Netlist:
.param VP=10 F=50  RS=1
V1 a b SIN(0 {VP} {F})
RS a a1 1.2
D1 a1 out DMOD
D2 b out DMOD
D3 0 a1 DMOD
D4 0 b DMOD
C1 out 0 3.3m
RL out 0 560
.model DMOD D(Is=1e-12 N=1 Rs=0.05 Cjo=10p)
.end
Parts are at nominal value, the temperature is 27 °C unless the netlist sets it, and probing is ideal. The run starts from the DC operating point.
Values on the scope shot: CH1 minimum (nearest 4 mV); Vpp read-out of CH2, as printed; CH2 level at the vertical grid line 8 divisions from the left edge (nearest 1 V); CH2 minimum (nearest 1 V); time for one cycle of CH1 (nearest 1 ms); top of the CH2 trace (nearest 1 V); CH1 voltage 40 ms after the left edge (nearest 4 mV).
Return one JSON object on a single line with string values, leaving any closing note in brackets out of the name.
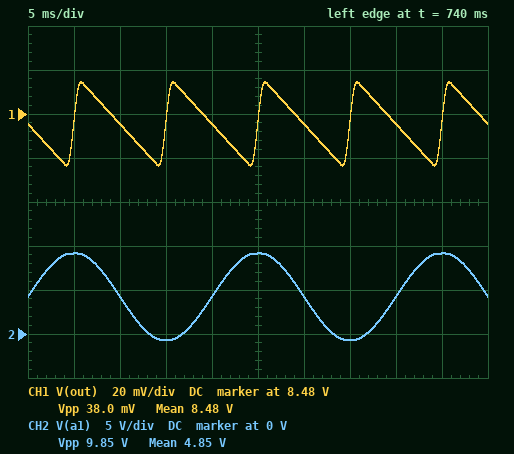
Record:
{"CH1 minimum": "8.456 V", "Vpp read-out of CH2, as printed": "9.85 V", "CH2 level at the vertical grid line 8 divisions from the left edge": "4 V", "CH2 minimum": "-1 V", "time for one cycle of CH1": "10 ms", "top of the CH2 trace": "9 V", "CH1 voltage 40 ms after the left edge": "8.476 V"}
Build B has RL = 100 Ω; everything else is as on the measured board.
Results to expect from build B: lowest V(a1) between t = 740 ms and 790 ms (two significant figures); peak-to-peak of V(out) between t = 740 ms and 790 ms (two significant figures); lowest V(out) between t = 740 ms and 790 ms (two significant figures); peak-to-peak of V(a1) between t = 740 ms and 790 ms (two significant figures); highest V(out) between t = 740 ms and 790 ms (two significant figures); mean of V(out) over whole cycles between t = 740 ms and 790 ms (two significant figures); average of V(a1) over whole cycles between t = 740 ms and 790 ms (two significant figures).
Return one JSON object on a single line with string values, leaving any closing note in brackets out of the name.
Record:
{"lowest V(a1) between t = 740 ms and 790 ms": "-720 mV", "peak-to-peak of V(out) between t = 740 ms and 790 ms": "180 mV", "lowest V(out) between t = 740 ms and 790 ms": "7.9 V", "peak-to-peak of V(a1) between t = 740 ms and 790 ms": "9.5 V", "highest V(out) between t = 740 ms and 790 ms": "8.1 V", "mean of V(out) over whole cycles between t = 740 ms and 790 ms": "8.0 V", "average of V(a1) over whole cycles between t = 740 ms and 790 ms": "4.0 V"}
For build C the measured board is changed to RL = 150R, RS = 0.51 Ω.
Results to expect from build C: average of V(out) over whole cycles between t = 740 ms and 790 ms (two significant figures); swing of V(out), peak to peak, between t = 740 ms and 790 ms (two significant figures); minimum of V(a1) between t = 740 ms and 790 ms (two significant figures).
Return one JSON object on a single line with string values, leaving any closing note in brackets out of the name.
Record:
{"average of V(out) over whole cycles between t = 740 ms and 790 ms": "8.3 V", "swing of V(out), peak to peak, between t = 740 ms and 790 ms": "140 mV", "minimum of V(a1) between t = 740 ms and 790 ms": "-720 mV"}
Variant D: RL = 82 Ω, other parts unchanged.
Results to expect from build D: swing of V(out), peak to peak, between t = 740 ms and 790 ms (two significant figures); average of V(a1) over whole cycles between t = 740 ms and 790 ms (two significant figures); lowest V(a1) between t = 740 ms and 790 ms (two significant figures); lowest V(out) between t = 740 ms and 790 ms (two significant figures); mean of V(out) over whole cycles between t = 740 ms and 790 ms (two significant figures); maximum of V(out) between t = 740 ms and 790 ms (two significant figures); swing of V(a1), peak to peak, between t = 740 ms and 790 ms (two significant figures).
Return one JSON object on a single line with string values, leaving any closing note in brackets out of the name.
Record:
{"swing of V(out), peak to peak, between t = 740 ms and 790 ms": "220 mV", "average of V(a1) over whole cycles between t = 740 ms and 790 ms": "3.9 V", "lowest V(a1) between t = 740 ms and 790 ms": "-730 mV", "lowest V(out) between t = 740 ms and 790 ms": "7.8 V", "mean of V(out) over whole cycles between t = 740 ms and 790 ms": "7.9 V", "maximum of V(out) between t = 740 ms and 790 ms": "8.0 V", "swing of V(a1), peak to peak, between t = 740 ms and 790 ms": "9.4 V"}
